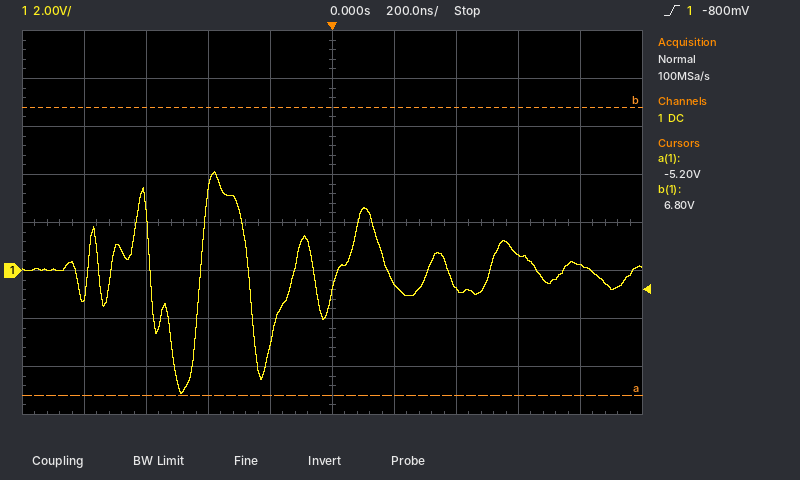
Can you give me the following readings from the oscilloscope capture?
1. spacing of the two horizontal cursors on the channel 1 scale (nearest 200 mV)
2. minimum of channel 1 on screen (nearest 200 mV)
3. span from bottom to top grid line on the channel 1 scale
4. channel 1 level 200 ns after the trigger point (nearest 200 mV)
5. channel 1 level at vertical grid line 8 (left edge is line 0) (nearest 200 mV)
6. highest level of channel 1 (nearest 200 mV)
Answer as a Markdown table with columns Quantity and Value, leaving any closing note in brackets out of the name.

| Quantity | Value |
|---|---|
| spacing of the two horizontal cursors on the channel 1 scale | 12.0 V |
| minimum of channel 1 on screen | -5.2 V |
| span from bottom to top grid line on the channel 1 scale | 16 V |
| channel 1 level 200 ns after the trigger point | -600 mV |
| channel 1 level at vertical grid line 8 (left edge is line 0) | 600 mV |
| highest level of channel 1 | 4.2 V |
